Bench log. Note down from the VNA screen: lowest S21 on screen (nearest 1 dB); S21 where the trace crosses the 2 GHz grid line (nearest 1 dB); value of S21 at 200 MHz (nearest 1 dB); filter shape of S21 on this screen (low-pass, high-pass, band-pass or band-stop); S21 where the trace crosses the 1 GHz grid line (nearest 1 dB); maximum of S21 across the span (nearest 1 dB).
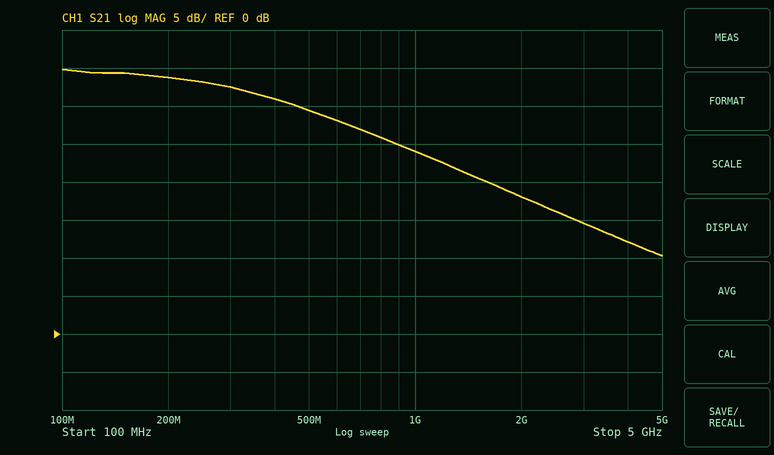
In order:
10 dB
18 dB
34 dB
low-pass
24 dB
35 dB
